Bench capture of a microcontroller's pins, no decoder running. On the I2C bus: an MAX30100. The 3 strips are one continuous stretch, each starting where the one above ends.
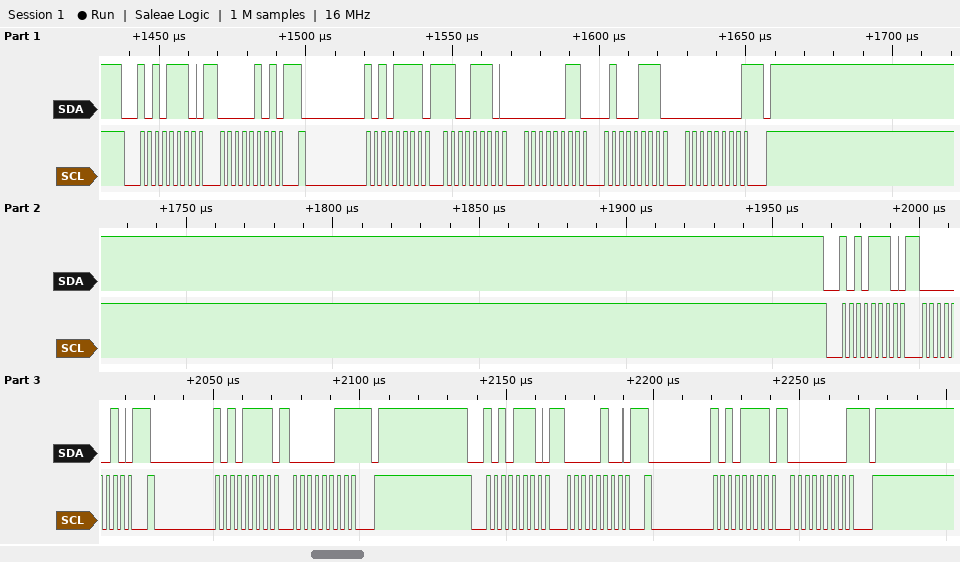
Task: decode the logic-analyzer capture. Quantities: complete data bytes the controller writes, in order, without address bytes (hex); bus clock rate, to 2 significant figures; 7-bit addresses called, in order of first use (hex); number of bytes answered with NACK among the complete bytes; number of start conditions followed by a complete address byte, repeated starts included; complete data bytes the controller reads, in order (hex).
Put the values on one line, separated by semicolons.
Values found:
05 02 04; 400 kHz; 0x57; 3; 6; CE 03 47 00 03 00
